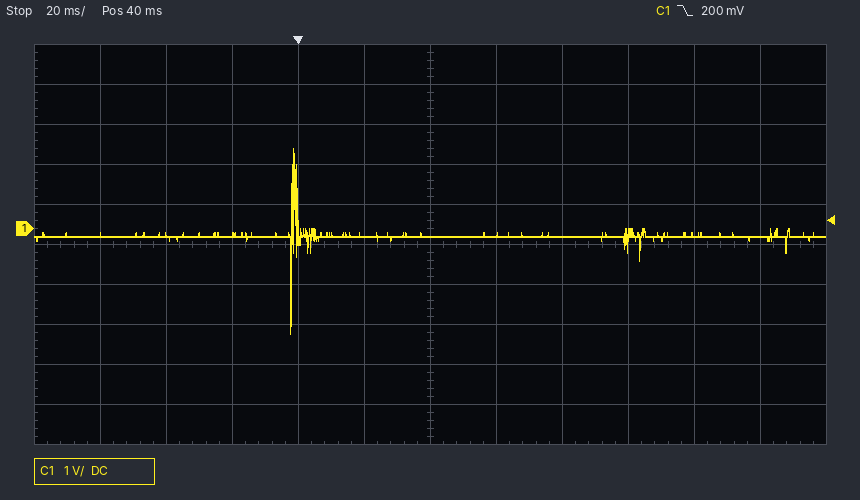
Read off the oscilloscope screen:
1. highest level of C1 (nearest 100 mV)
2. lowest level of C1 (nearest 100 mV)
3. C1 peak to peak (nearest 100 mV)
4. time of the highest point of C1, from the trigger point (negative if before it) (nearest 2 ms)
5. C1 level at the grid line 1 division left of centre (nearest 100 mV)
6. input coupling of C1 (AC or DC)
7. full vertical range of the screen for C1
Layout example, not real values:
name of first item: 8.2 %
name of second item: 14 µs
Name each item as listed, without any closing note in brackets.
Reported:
highest level of C1: 2.0 V
lowest level of C1: -2.6 V
C1 peak to peak: 4.6 V
time of the highest point of C1, from the trigger point (negative if before it): -2 ms
C1 level at the grid line 1 division left of centre: -200 mV
input coupling of C1: DC
full vertical range of the screen for C1: 10 V
